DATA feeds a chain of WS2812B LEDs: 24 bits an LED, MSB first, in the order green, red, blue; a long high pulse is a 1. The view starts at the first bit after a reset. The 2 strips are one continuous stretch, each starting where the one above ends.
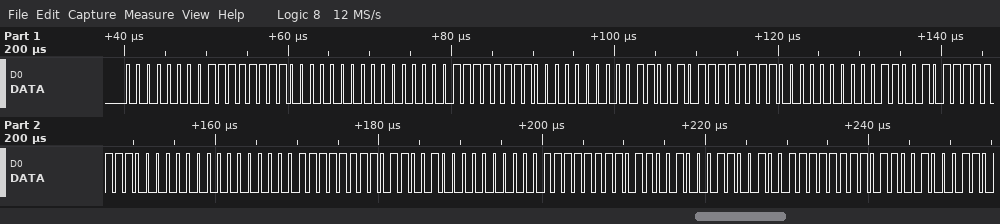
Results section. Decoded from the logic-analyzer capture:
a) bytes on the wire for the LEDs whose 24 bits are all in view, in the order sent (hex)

00 FF 00 00 FF 00 32 FF 00 32 FF 00 00 FF 64 00 FF 64 64 FF 64
